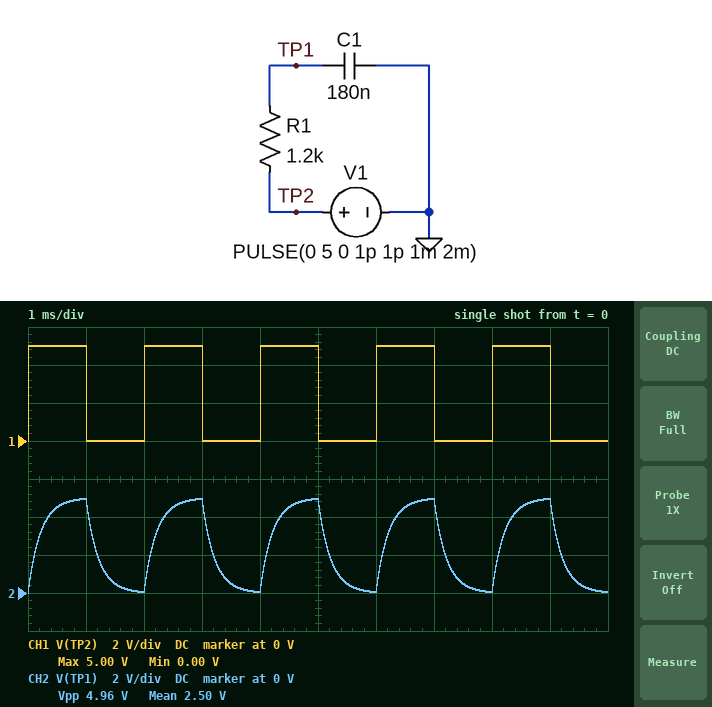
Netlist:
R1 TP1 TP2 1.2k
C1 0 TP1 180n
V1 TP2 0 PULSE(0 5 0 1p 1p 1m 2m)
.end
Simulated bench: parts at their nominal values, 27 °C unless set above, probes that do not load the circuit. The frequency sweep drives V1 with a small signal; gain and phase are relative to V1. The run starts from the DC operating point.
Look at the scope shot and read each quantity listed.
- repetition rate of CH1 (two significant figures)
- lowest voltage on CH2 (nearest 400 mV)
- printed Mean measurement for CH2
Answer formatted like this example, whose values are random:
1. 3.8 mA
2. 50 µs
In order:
1. 500 Hz
2. 0 V
3. 2.50 V
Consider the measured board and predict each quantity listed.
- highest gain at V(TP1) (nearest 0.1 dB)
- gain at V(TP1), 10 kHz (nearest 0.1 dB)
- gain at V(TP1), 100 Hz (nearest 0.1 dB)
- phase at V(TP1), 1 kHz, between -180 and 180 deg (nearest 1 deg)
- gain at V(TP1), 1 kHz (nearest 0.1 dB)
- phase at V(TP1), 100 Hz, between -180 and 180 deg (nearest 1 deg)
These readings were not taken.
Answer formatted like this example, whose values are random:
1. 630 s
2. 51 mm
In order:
1. 0 dB
2. -22.7 dB
3. -0.1 dB
4. -54 deg
5. -4.5 dB
6. -8 deg
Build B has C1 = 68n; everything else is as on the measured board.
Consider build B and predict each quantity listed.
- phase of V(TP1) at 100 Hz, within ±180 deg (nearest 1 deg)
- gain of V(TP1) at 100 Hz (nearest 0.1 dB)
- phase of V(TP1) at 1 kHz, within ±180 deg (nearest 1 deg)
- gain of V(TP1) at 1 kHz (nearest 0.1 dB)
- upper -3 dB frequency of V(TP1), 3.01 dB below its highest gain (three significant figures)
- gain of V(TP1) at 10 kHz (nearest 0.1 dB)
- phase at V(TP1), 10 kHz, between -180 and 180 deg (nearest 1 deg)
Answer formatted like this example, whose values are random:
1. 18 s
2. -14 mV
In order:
1. -3 deg
2. 0 dB
3. -27 deg
4. -1.0 dB
5. 1.95 kHz
6. -14.4 dB
7. -79 deg
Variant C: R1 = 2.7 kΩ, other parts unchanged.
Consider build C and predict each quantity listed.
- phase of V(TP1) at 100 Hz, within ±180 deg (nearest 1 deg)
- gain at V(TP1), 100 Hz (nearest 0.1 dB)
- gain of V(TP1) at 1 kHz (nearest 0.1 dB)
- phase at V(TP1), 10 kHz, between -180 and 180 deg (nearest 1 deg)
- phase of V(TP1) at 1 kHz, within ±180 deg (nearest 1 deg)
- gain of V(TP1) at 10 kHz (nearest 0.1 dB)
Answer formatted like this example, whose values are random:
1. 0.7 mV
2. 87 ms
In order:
1. -17 deg
2. -0.4 dB
3. -10.1 dB
4. -88 deg
5. -72 deg
6. -29.7 dB
